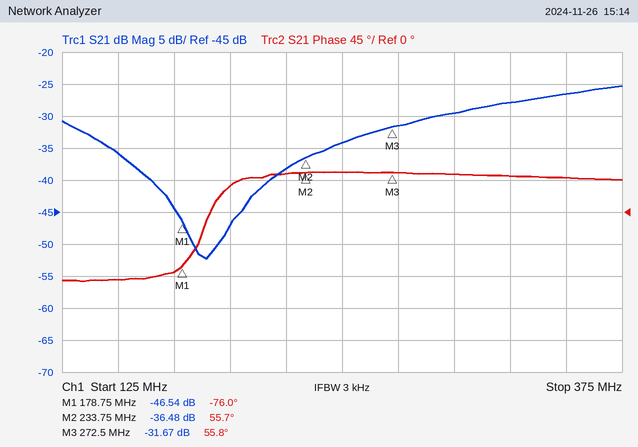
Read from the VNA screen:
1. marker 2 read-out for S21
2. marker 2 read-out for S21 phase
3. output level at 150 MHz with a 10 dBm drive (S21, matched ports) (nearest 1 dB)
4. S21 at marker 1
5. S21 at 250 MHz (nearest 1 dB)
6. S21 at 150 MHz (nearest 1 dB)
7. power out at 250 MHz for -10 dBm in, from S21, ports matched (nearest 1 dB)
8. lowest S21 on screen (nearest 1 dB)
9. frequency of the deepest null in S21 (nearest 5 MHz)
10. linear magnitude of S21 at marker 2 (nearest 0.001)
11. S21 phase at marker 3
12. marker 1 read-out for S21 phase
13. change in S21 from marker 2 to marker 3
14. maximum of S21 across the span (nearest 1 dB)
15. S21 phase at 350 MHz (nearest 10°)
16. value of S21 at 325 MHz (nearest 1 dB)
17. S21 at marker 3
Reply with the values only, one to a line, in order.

-36.48 dB
55.7°
-26 dBm
-46.54 dB
-34 dB
-36 dB
-44 dBm
-52 dB
190 MHz
0.015
55.8°
-76.0°
4.81 dB
-25 dB
50°
-28 dB
-31.67 dB
